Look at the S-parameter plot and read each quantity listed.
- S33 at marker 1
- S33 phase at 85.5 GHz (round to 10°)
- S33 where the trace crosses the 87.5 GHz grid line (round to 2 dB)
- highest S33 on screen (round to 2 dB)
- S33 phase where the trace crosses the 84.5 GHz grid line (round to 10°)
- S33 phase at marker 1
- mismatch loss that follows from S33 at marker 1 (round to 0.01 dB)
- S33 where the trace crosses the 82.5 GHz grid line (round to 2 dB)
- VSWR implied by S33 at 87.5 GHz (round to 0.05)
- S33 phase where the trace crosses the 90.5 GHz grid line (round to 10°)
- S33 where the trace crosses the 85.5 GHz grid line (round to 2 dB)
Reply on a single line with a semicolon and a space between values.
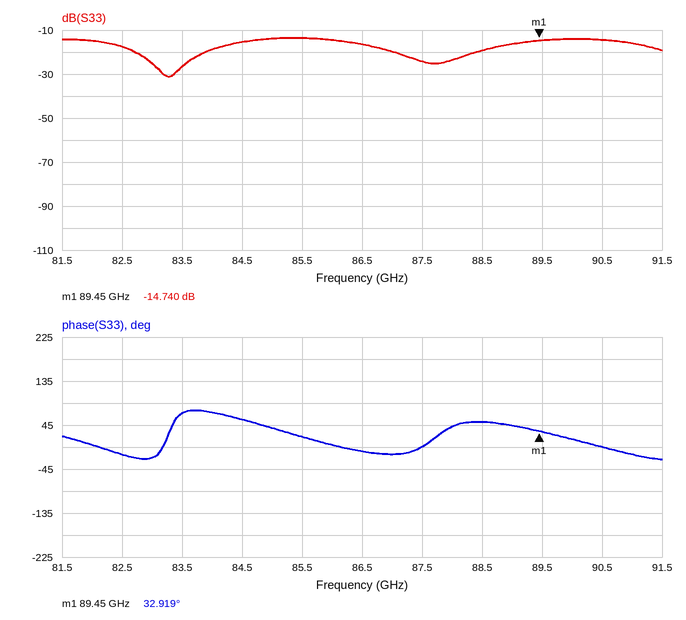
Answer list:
-14.740 dB; 20°; -24 dB; -14 dB; 60°; 32.919°; 0.15 dB; -18 dB; 1.15; 0°; -14 dB
